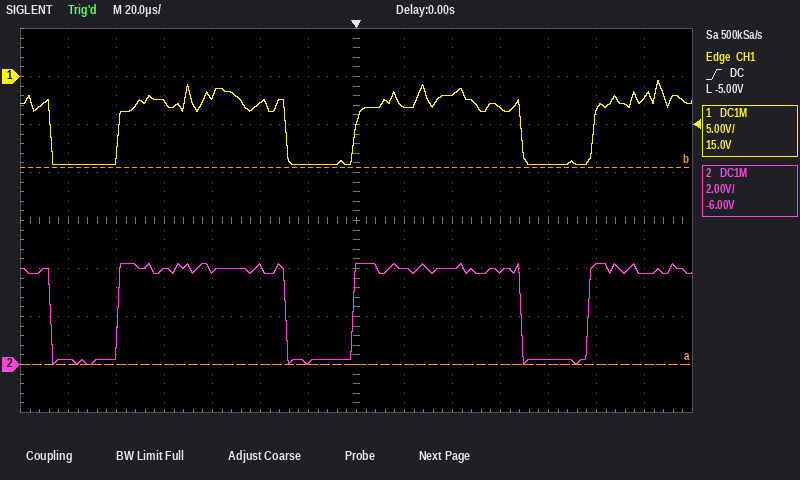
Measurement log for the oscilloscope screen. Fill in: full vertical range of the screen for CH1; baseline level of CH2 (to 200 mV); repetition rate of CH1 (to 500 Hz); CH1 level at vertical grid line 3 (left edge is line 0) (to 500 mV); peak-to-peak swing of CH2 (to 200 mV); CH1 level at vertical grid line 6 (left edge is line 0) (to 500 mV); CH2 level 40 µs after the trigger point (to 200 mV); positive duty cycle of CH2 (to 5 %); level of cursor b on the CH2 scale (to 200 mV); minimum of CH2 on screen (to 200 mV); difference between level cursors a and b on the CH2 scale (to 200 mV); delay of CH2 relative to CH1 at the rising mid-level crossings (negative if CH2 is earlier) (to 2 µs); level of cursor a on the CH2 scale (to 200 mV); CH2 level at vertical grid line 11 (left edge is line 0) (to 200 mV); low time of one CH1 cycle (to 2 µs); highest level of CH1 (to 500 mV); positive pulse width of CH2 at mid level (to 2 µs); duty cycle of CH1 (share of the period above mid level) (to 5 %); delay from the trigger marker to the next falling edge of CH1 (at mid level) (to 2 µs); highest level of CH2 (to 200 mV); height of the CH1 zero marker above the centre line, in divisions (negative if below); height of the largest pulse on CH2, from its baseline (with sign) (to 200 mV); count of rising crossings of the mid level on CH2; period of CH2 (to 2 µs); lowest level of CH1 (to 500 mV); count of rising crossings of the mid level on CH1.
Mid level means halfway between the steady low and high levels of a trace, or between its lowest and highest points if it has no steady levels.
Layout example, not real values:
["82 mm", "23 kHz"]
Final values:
["40 V", "4.0 V", "10.0 kHz", "-2.5 V", "4.2 V", "-9.0 V", "4.0 V", "70 %", "8.2 V", "0.0 V", "8.2 V", "-2 µs", "0.0 V", "200 mV", "30 µs", "-500 mV", "70 µs", "70 %", "68 µs", "4.2 V", "+3.0 div", "-4.0 V", "3", "98 µs", "-9.0 V", "3"]
